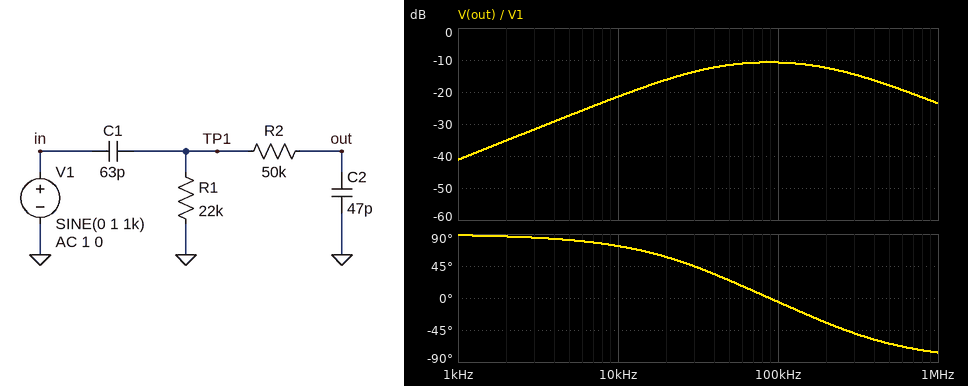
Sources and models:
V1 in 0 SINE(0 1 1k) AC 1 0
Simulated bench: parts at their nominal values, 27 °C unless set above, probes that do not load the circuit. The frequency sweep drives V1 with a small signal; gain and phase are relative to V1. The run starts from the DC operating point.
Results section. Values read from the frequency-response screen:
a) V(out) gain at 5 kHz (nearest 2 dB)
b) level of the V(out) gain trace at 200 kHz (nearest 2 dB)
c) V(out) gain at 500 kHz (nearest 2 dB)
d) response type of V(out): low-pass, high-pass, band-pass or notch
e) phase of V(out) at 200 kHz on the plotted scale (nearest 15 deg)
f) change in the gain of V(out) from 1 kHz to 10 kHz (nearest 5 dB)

-28 dB
-12 dB
-18 dB
band-pass
-30 deg
20 dB
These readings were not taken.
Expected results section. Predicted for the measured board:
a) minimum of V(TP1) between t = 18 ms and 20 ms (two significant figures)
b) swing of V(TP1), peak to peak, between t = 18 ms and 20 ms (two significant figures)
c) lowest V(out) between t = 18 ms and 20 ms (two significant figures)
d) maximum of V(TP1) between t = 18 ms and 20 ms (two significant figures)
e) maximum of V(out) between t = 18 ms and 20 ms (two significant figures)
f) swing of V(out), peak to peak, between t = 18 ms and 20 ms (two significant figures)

-8.7 mV
17 mV
-8.7 mV
8.7 mV
8.7 mV
17 mV
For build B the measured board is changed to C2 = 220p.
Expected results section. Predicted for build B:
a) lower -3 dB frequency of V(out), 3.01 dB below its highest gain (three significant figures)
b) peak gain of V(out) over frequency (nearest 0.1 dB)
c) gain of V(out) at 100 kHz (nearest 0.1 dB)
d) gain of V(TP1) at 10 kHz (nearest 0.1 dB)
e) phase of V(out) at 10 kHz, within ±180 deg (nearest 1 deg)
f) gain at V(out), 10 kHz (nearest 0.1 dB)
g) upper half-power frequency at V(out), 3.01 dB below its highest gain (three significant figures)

8.81 kHz
-21.9 dB
-22.7 dB
-22.6 dB
41 deg
-24.3 dB
189 kHz
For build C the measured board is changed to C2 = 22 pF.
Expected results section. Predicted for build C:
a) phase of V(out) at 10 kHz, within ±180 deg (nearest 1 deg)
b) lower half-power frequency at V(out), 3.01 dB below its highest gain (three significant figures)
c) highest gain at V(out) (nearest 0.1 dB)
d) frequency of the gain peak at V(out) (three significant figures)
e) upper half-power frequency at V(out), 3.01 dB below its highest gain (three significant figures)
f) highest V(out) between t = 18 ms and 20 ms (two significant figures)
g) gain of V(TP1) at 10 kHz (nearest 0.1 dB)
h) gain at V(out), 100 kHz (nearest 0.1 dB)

79 deg
46.6 kHz
-6.6 dB
129 kHz
357 kHz
8.7 mV
-21.3 dB
-6.8 dB
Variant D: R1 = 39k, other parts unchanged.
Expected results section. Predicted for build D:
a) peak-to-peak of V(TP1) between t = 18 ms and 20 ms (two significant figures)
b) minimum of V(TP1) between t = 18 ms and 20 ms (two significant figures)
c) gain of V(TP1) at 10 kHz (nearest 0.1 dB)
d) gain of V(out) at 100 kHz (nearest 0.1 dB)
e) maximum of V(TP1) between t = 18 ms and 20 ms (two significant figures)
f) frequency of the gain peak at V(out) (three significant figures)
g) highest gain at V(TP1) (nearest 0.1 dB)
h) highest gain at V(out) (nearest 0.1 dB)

31 mV
-15 mV
-16.7 dB
-9.0 dB
15 mV
66.2 kHz
0 dB
-8.6 dB
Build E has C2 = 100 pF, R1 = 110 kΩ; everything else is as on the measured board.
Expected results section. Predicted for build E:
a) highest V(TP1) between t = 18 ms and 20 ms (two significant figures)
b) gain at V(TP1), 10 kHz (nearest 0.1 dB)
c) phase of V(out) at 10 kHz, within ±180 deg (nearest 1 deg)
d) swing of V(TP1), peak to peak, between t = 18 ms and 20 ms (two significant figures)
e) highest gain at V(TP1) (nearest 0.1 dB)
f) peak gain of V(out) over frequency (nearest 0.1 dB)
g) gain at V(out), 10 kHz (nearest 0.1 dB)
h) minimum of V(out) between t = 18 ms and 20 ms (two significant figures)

43 mV
-11.3 dB
31 deg
86 mV
0 dB
-10.4 dB
-11.7 dB
-43 mV
